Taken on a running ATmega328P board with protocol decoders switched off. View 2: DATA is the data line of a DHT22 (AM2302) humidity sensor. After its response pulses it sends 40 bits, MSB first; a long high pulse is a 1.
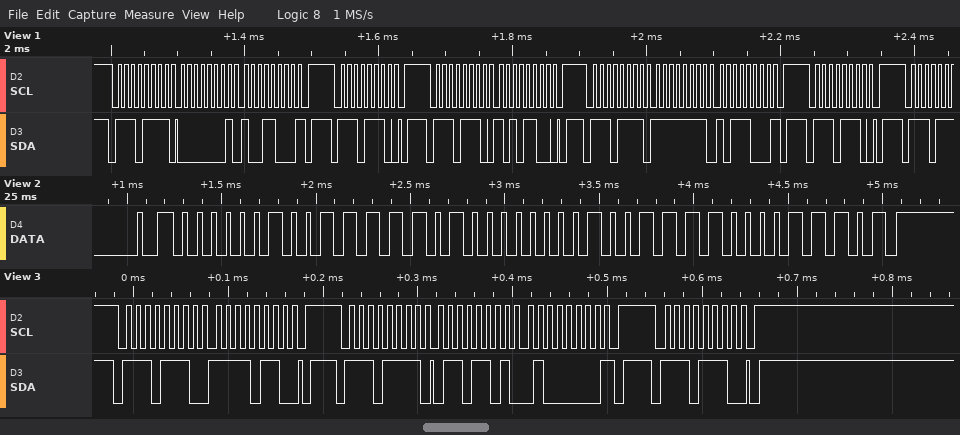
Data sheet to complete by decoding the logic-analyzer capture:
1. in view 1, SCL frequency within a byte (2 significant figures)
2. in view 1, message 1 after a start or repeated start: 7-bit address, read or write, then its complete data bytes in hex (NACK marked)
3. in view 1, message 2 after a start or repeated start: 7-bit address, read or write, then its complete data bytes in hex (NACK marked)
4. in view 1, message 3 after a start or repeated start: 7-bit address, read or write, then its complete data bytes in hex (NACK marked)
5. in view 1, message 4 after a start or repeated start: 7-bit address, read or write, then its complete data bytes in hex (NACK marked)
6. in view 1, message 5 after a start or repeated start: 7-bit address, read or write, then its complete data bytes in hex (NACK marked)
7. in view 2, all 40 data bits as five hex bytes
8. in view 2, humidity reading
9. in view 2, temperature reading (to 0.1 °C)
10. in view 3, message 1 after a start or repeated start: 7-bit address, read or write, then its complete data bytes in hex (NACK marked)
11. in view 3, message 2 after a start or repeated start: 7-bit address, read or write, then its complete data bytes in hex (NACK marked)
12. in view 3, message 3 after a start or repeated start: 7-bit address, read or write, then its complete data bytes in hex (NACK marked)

100 kHz
0x77 read: 01 98 NACK
0x77 write
0x77 write: AC
0x77 read: FF B8 NACK
0x77 write
02 7D 00 9E 1D
63.7 %
15.8 °C
0x77 write: F6
0x77 read: 6D 40 NACK
0x77 write
